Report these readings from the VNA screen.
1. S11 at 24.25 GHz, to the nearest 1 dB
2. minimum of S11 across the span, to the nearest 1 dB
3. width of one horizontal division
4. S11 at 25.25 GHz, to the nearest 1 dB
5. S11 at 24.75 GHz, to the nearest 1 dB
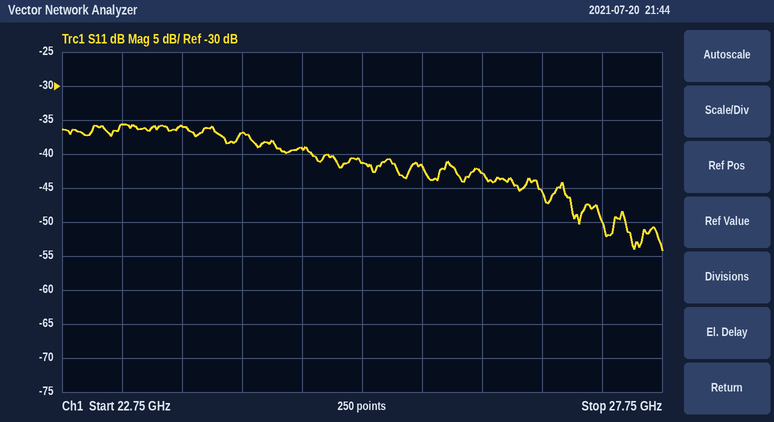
-37 dB
-54 dB
500 MHz
-41 dB
-39 dB
